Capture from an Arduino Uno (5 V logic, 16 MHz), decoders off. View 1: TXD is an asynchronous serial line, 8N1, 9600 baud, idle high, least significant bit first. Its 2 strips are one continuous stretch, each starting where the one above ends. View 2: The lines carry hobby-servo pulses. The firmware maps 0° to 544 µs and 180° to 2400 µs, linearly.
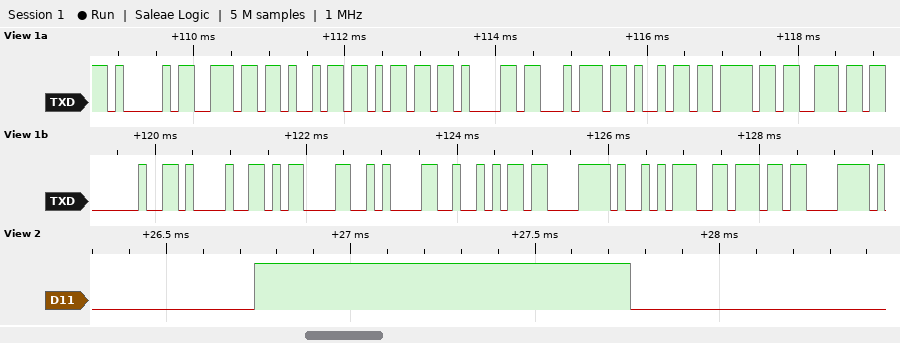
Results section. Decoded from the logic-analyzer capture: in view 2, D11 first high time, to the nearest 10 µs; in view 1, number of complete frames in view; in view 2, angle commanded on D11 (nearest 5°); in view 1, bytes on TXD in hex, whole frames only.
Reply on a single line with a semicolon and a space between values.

1020 µs; 18; 45°; 41 6E 69 6D 61 74 69 6F 6E 20 21 0D 0A 52 C3 A9 76 C3
